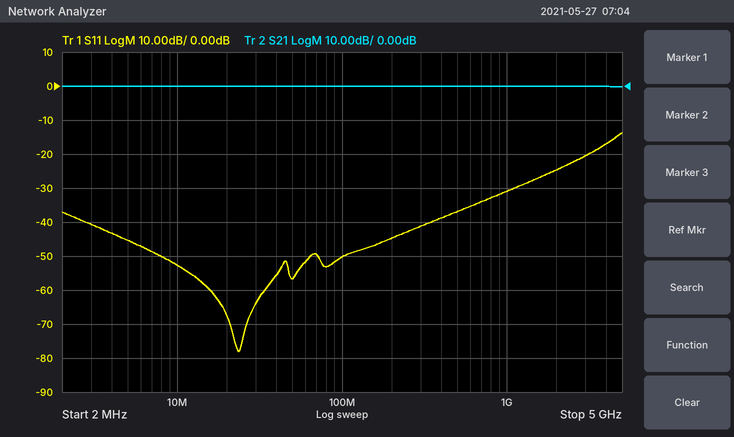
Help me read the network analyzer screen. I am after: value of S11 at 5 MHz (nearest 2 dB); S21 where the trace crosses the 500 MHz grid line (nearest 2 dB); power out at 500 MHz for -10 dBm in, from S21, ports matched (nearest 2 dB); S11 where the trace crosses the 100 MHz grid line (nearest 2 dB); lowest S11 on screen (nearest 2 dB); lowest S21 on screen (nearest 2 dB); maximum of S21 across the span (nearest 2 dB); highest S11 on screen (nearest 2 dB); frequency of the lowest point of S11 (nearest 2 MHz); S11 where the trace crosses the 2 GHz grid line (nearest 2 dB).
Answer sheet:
-46 dB
0 dB
-10 dBm
-50 dB
-78 dB
0 dB
0 dB
-14 dB
24 MHz
-24 dB
